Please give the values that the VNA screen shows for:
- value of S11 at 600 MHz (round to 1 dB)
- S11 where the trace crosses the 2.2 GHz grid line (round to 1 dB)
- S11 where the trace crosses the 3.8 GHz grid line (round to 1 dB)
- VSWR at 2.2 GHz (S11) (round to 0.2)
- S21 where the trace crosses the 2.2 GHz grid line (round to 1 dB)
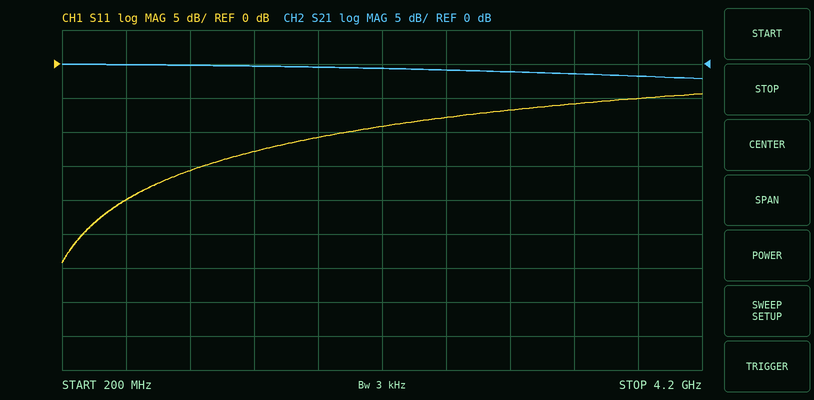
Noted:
-20 dB
-9 dB
-5 dB
2.0
-1 dB
